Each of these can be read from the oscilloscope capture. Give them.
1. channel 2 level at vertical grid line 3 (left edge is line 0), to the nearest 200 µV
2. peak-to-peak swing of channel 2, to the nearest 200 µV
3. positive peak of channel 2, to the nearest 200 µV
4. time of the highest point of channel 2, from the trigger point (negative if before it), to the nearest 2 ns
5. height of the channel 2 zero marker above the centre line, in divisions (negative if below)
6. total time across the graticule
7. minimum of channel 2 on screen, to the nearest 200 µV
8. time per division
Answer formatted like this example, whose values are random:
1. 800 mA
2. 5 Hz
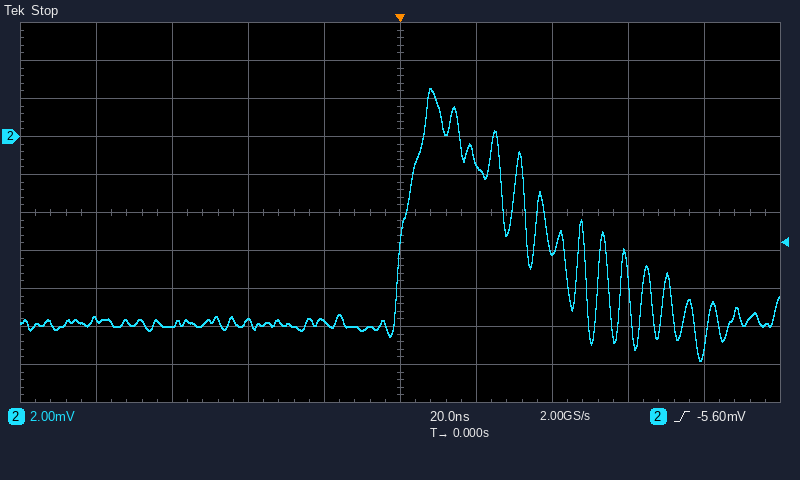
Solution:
1. -9.8 mV
2. 14.4 mV
3. 2.6 mV
4. +8 ns
5. +2.0 div
6. 200 ns
7. -11.8 mV
8. 20 ns
